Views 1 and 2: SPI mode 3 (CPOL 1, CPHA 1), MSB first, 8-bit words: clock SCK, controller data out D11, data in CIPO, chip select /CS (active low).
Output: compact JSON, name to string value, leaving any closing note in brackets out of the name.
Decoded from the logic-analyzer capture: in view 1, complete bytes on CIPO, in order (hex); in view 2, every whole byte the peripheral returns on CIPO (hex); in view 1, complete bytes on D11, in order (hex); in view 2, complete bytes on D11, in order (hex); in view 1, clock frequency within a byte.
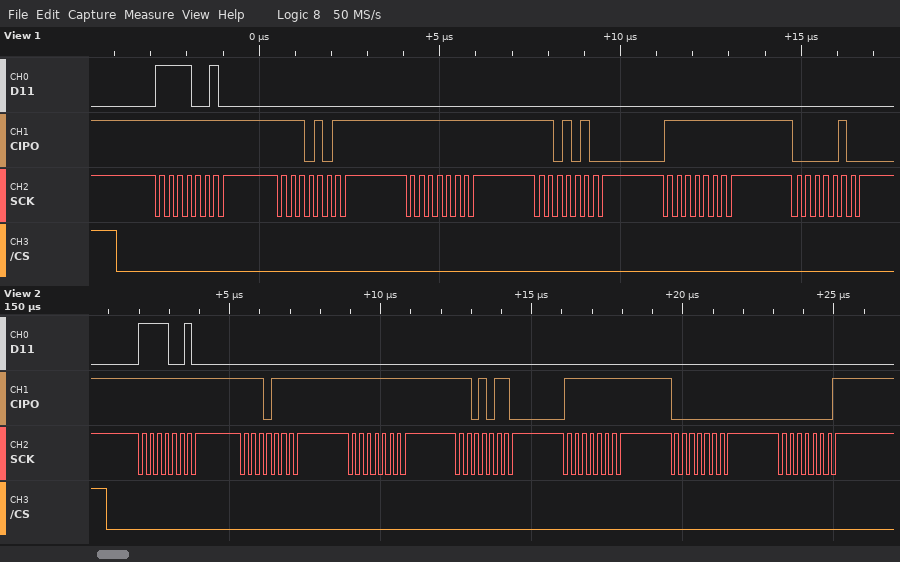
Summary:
{"in view 1, complete bytes on CIPO, in order": "FF EB FF D4 FF 04", "in view 2, every whole byte the peripheral returns on CIPO": "FF EF FF D6 FF 00 01", "in view 1, complete bytes on D11, in order": "F2 00 00 00 00 00", "in view 2, complete bytes on D11, in order": "F2 00 00 00 00 00 00", "in view 1, clock frequency within a byte": "4 MHz"}
